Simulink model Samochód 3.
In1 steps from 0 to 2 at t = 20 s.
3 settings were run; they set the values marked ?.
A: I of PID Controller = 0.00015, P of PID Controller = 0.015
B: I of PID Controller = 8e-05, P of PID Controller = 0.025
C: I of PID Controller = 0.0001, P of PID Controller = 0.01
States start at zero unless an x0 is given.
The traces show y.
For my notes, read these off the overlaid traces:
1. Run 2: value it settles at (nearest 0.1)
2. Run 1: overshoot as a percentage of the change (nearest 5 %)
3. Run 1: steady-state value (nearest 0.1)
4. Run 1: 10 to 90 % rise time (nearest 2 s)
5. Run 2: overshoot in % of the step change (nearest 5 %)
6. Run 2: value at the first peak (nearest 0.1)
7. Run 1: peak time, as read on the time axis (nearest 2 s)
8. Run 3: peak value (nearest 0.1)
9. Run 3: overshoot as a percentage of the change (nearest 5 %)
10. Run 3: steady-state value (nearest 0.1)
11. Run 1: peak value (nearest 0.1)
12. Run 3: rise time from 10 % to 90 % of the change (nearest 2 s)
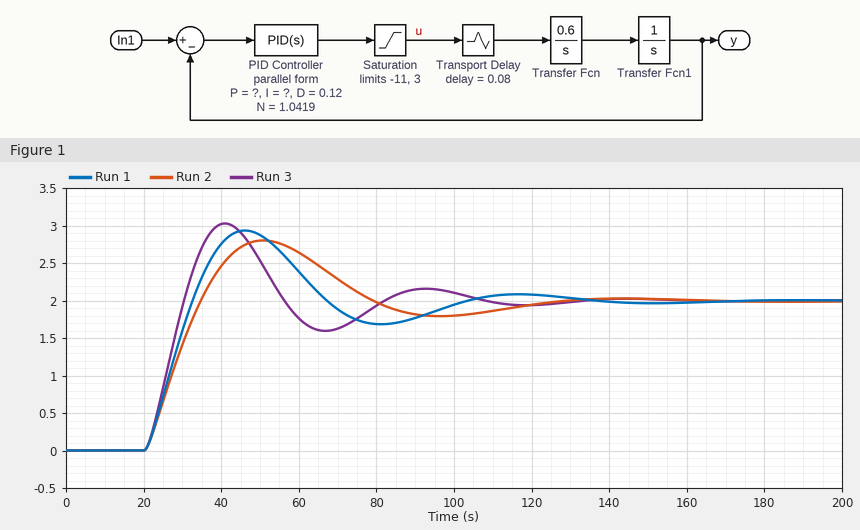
2.0
45 %
2.0
10 s
40 %
2.8
46 s
3.0
50 %
2.0
2.9
8 s
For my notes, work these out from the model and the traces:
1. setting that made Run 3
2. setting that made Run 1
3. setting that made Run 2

B
A
C
